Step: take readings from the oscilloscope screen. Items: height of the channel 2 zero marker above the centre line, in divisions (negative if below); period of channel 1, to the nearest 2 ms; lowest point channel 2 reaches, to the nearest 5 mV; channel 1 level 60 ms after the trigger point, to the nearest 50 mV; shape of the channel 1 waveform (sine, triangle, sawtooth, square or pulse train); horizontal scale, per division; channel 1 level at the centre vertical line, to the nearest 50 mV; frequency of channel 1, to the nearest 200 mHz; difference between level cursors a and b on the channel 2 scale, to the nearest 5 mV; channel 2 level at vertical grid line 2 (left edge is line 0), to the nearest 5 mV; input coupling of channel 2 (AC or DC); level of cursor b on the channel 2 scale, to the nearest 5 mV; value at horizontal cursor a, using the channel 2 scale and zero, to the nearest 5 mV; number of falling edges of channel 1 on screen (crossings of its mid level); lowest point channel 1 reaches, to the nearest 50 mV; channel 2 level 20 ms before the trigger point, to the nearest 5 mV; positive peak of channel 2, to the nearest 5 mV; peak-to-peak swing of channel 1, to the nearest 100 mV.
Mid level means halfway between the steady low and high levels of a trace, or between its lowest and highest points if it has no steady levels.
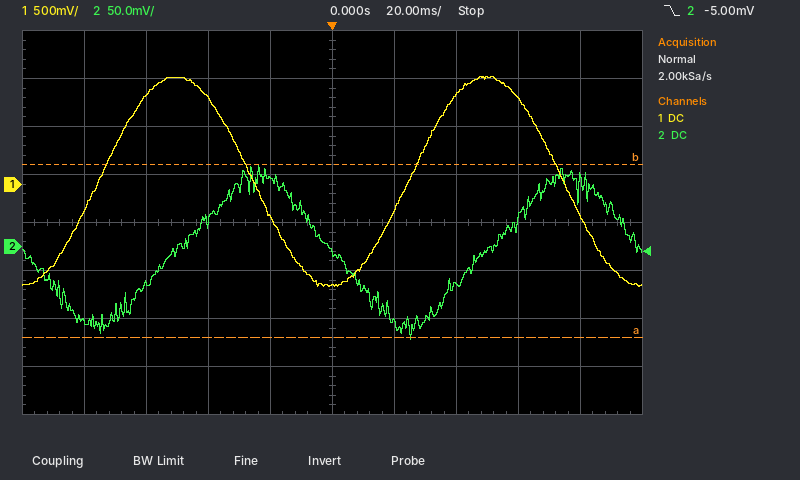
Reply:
-0.5 div
100 ms
-95 mV
900 mV
sine
20 ms
-1.05 V
10.0 Hz
180 mV
-40 mV
DC
85 mV
-95 mV
2
-1.05 V
70 mV
85 mV
2.20 V
